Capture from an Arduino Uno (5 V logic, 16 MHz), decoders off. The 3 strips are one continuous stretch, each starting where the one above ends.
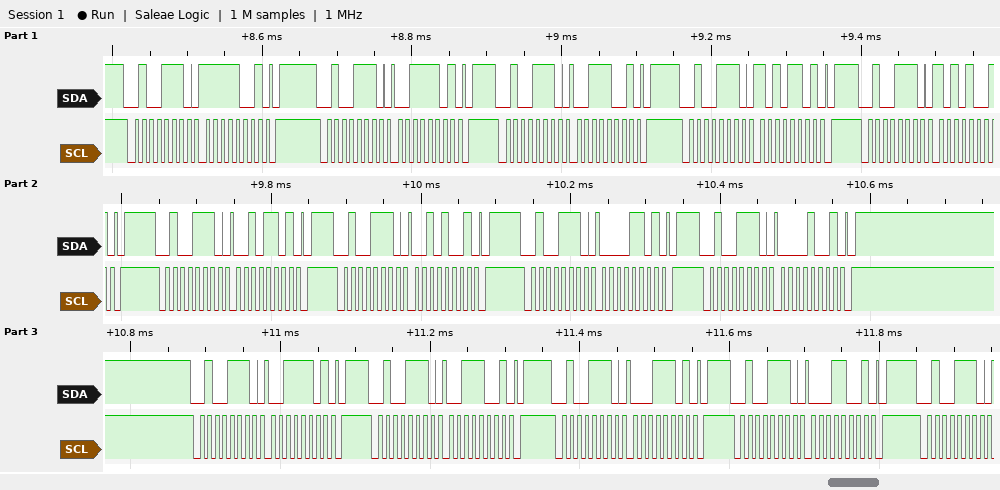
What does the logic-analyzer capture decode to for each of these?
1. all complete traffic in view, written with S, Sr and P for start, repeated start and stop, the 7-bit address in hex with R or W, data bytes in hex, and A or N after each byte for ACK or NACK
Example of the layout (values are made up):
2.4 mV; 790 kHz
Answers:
S 27W A F9 A P S 27W A 3D A P S 27W A 39 A P S 27W A AD A P S 27W A A9 A P S 27W A 2D A P S 27W A 29 A P S 27W A 0D A P S 27W A 09 A P S 27W A 3D A P S 27W A 39 A P S 27W A 1D A P S 27W A 19 A P S 27W A
